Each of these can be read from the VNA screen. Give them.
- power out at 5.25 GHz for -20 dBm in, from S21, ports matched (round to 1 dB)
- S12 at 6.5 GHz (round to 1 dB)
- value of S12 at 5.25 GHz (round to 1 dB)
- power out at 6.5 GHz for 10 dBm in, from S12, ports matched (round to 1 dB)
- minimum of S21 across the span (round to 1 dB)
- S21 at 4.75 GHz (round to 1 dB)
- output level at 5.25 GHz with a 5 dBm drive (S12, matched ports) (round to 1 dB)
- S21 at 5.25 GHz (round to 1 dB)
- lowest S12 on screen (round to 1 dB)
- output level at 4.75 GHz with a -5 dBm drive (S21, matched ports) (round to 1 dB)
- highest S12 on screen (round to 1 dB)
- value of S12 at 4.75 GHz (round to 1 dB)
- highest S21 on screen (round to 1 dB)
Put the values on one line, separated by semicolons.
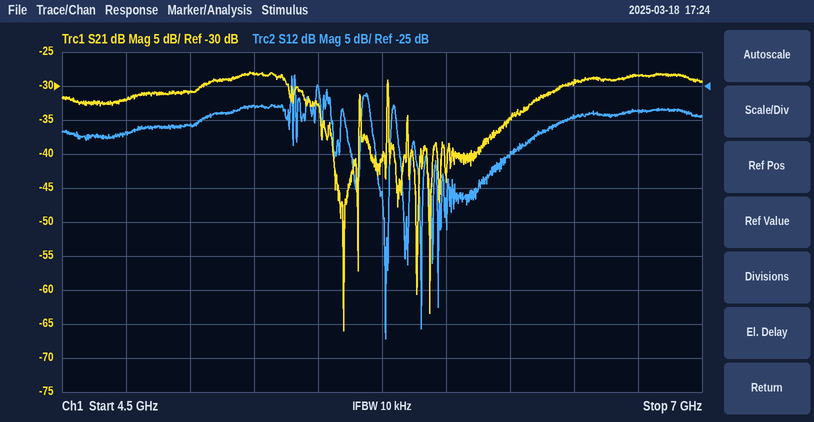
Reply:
-48 dBm; -30 dB; -28 dB; -20 dBm; -66 dB; -32 dB; -23 dBm; -28 dB; -62 dB; -37 dBm; -23 dB; -32 dB; -28 dB
